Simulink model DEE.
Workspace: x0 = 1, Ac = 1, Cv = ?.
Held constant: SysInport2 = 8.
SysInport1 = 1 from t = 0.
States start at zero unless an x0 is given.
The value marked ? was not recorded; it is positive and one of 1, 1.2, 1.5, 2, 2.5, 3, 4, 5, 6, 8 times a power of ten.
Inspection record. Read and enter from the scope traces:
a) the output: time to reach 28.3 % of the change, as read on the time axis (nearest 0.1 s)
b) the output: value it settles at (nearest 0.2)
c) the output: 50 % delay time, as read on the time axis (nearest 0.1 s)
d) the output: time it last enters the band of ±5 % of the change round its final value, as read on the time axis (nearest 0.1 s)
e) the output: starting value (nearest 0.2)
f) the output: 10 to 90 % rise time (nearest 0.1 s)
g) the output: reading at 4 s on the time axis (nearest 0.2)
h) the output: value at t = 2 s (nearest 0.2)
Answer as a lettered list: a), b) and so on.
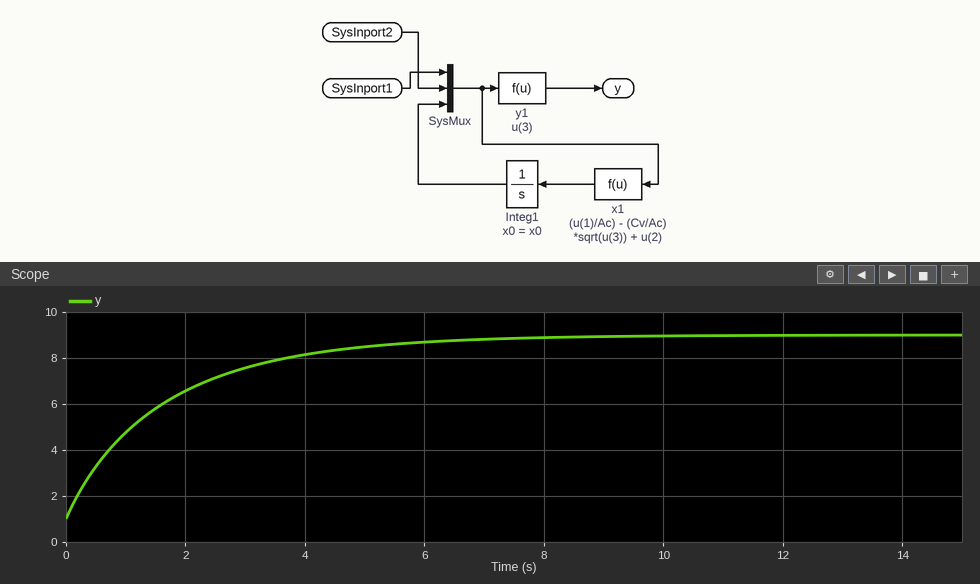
a) 0.5 s
b) 9.0
c) 1.1 s
d) 5.5 s
e) 1.0
f) 4.0 s
g) 8.2
h) 6.6
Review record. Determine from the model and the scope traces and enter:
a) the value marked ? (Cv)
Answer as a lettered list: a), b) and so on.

a) 3
